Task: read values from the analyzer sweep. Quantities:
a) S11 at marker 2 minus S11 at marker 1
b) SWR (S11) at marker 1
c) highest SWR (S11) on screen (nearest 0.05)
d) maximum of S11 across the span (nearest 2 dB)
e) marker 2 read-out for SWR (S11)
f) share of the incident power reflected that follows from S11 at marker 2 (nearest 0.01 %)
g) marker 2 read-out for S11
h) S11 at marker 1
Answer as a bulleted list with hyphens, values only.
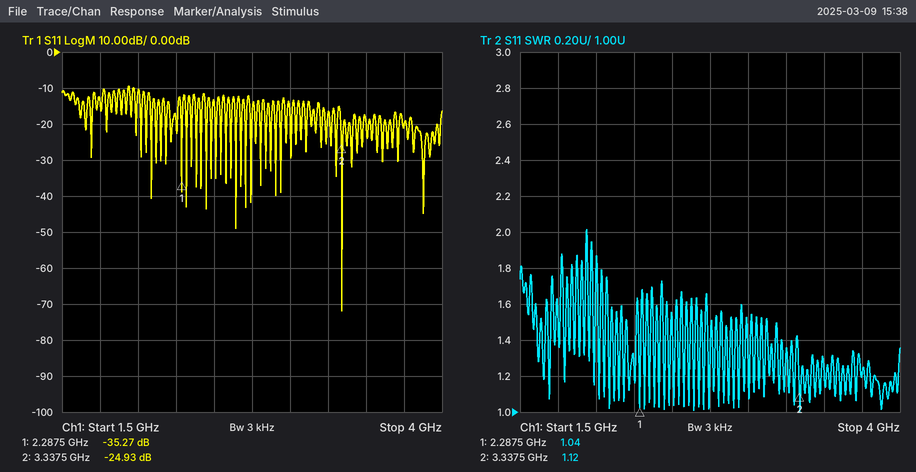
- 10.34 dB
- 1.04
- 2.00
- -10 dB
- 1.12
- 0.32 %
- -24.93 dB
- -35.27 dB
